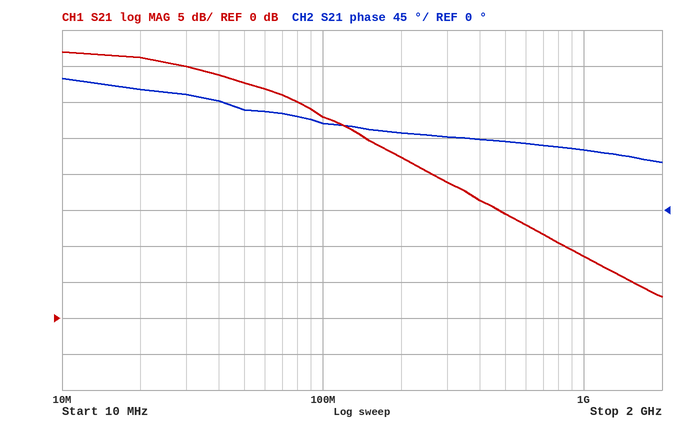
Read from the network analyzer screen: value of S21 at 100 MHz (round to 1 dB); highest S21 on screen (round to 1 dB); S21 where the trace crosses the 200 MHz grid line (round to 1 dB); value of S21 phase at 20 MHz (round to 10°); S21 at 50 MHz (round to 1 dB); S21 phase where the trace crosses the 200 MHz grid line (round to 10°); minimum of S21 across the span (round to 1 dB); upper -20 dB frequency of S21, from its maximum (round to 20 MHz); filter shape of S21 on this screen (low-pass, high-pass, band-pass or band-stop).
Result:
28 dB
37 dB
22 dB
150°
33 dB
100°
3 dB
380 MHz
low-pass
